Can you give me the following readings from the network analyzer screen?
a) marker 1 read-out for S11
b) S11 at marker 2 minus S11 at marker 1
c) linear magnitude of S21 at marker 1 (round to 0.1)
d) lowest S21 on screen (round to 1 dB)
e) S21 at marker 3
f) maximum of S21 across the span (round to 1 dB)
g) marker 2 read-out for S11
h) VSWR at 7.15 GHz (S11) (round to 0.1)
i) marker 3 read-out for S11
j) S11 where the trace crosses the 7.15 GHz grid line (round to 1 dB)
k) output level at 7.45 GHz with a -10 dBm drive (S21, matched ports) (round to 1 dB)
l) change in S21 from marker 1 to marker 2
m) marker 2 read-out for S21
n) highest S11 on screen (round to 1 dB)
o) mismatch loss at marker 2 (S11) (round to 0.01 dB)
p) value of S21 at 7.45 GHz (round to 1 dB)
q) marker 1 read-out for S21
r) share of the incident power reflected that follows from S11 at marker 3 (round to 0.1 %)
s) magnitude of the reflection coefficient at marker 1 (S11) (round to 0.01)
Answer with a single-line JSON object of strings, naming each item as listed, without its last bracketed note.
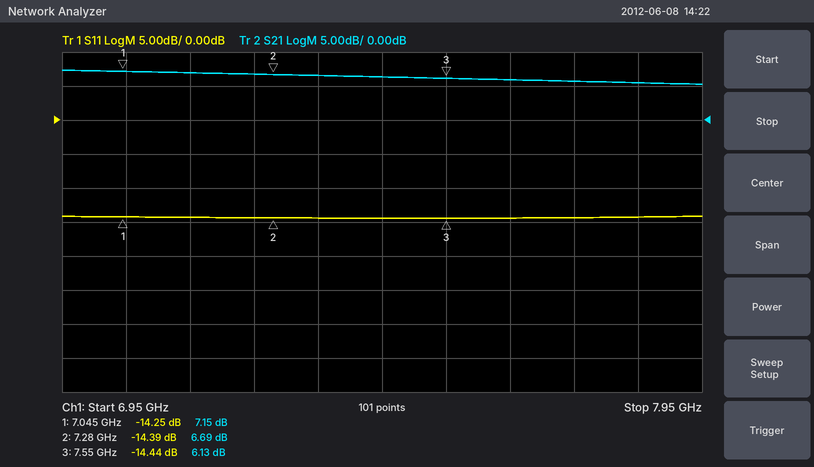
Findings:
{"marker 1 read-out for S11": "-14.25 dB", "S11 at marker 2 minus S11 at marker 1": "-0.14 dB", "linear magnitude of S21 at marker 1": "2.3", "lowest S21 on screen": "5 dB", "S21 at marker 3": "6.13 dB", "maximum of S21 across the span": "7 dB", "marker 2 read-out for S11": "-14.39 dB", "VSWR at 7.15 GHz (S11)": "1.5", "marker 3 read-out for S11": "-14.44 dB", "S11 where the trace crosses the 7.15 GHz grid line": "-14 dB", "output level at 7.45 GHz with a -10 dBm drive (S21, matched ports)": "-4 dBm", "change in S21 from marker 1 to marker 2": "-0.46 dB", "marker 2 read-out for S21": "6.69 dB", "highest S11 on screen": "-14 dB", "mismatch loss at marker 2 (S11)": "0.16 dB", "value of S21 at 7.45 GHz": "6 dB", "marker 1 read-out for S21": "7.15 dB", "share of the incident power reflected that follows from S11 at marker 3": "3.6 %", "magnitude of the reflection coefficient at marker 1 (S11)": "0.19"}
